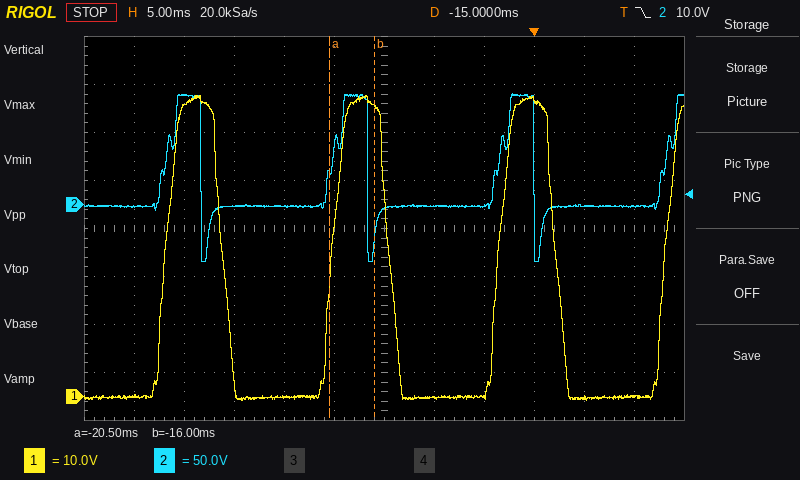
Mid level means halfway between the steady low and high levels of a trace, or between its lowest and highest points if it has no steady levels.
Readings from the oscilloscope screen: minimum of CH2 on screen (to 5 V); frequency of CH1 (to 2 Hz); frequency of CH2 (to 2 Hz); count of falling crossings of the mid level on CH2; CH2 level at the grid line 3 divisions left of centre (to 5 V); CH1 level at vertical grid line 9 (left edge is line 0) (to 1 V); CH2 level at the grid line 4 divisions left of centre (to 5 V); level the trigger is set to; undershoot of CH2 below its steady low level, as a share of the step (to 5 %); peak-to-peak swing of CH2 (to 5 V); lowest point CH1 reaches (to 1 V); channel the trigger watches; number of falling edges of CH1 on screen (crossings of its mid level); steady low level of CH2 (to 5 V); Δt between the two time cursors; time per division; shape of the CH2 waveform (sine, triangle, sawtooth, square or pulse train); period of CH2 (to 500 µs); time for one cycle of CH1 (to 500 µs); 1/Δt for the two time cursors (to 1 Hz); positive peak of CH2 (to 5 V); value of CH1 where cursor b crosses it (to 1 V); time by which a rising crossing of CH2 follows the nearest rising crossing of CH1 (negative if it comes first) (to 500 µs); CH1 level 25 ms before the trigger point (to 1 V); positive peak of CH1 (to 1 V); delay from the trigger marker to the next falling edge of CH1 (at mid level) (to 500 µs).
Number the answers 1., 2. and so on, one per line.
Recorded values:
1. -60 V
2. 60 Hz
3. 60 Hz
4. 3
5. 0 V
6. 62 V
7. 115 V
8. 10.0 V
9. 50 %
10. 175 V
11. -1 V
12. CH2
13. 3
14. 0 V
15. 4.5 ms
16. 5 ms
17. pulse train
18. 16.5 ms
19. 16.5 ms
20. 222 Hz
21. 115 V
22. 60 V
23. 0.0 ms
24. 0 V
25. 63 V
26. 2.0 ms
